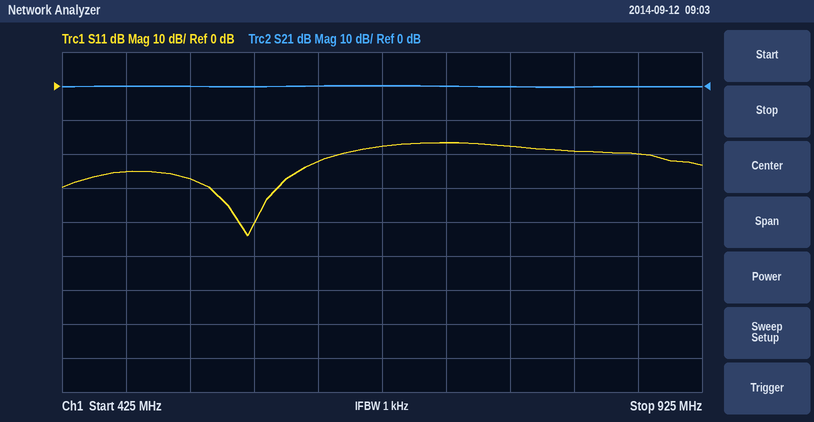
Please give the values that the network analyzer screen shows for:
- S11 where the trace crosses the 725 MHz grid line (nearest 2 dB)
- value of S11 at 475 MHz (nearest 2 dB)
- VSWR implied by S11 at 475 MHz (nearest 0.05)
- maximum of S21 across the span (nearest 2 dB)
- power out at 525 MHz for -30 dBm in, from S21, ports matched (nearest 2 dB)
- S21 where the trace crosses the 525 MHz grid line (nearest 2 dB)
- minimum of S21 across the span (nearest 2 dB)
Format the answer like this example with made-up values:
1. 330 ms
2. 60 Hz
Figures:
1. -16 dB
2. -26 dB
3. 1.10
4. 0 dB
5. -30 dBm
6. 0 dB
7. 0 dB
